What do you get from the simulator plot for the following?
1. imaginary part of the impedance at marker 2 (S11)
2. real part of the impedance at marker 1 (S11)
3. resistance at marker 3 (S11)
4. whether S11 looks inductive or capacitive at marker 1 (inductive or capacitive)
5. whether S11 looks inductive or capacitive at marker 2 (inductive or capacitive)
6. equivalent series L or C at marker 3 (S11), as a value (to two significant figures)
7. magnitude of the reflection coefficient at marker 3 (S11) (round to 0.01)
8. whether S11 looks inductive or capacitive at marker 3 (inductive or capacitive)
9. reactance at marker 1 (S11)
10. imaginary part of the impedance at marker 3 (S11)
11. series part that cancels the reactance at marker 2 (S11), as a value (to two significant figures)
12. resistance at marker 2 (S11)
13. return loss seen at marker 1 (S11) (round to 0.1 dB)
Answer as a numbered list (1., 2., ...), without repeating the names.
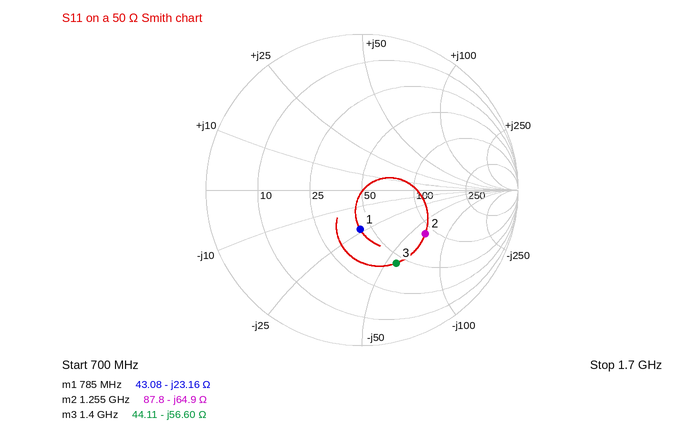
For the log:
1. -64.9 Ω
2. 43.08 Ω
3. 44.11 Ω
4. capacitive
5. capacitive
6. 2.0 pF
7. 0.52
8. capacitive
9. -23.16 Ω
10. -56.60 Ω
11. 8.2 nH
12. 87.8 Ω
13. 12.0 dB
